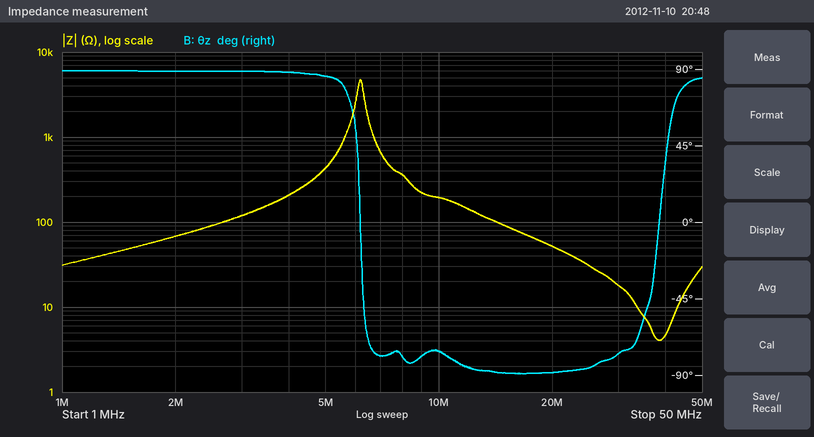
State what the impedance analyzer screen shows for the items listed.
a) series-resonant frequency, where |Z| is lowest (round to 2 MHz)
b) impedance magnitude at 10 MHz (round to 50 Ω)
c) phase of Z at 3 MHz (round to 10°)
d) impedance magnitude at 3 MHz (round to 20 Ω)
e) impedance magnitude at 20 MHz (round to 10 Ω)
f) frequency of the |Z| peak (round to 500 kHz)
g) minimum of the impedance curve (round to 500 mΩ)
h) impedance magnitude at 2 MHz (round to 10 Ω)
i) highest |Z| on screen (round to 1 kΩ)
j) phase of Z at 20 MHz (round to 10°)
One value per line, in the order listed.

38 MHz
200 Ω
90°
120 Ω
50 Ω
6.0 MHz
4.0 Ω
70 Ω
5 kΩ
-90°
